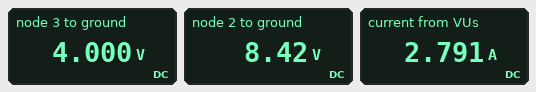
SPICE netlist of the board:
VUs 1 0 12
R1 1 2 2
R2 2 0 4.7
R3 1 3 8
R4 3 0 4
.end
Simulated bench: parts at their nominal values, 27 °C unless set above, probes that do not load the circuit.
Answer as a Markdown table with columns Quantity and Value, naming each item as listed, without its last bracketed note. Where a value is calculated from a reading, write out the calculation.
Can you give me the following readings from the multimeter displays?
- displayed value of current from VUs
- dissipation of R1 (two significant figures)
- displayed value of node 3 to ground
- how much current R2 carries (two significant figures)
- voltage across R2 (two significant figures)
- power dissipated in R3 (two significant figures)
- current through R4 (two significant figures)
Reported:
| Quantity | Value |
|---|---|
| displayed value of current from VUs | 2.791 A |
| dissipation of R1 | (12 V - 8.42 V)^2 / 2 Ω = 6.4 W |
| displayed value of node 3 to ground | 4.000 V |
| how much current R2 carries | (8.42 V) / 4.7 Ω = 1.8 A |
| voltage across R2 | 8.42 V = 8.4 V |
| power dissipated in R3 | (12 V - 4 V)^2 / 8 Ω = 8.0 W |
| current through R4 | (4 V) / 4 Ω = 1.0 A |
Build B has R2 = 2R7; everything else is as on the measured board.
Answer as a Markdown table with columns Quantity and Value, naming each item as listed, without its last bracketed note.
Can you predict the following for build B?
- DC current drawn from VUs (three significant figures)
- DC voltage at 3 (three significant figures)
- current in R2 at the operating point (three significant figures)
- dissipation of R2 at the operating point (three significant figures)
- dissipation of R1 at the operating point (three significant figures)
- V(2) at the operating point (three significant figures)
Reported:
| Quantity | Value |
|---|---|
| DC current drawn from VUs | 3.55 A |
| DC voltage at 3 | 4.00 V |
| current in R2 at the operating point | 2.55 A |
| dissipation of R2 at the operating point | 17.6 W |
| dissipation of R1 at the operating point | 13.0 W |
| V(2) at the operating point | 6.89 V |
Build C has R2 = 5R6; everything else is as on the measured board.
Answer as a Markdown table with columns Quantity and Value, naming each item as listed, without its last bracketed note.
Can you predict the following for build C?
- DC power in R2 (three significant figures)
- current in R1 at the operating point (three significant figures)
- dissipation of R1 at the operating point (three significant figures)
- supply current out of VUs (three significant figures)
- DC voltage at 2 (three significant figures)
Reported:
| Quantity | Value |
|---|---|
| DC power in R2 | 14.0 W |
| current in R1 at the operating point | 1.58 A |
| dissipation of R1 at the operating point | 4.99 W |
| supply current out of VUs | 2.58 A |
| DC voltage at 2 | 8.84 V |
